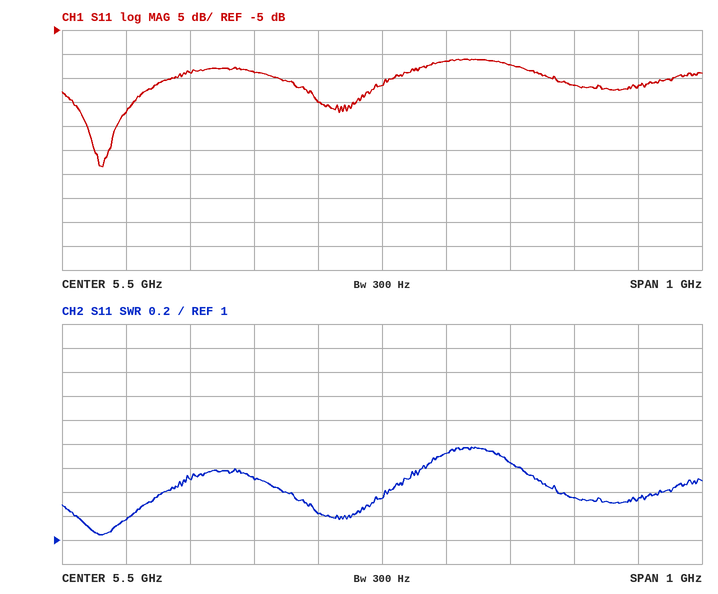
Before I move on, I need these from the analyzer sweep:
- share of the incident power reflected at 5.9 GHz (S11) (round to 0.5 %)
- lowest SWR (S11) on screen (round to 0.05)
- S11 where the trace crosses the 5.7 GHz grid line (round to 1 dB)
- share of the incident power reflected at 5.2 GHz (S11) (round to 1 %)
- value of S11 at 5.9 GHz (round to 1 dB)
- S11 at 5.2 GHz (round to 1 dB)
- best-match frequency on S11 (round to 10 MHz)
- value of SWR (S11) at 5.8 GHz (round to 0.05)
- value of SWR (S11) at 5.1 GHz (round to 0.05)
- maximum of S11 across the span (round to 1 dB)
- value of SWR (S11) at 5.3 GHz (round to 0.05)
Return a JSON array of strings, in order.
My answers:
["2.0 %", "1.05", "-12 dB", "4 %", "-17 dB", "-14 dB", "5.06 GHz", "1.35", "1.15", "-11 dB", "1.50"]
